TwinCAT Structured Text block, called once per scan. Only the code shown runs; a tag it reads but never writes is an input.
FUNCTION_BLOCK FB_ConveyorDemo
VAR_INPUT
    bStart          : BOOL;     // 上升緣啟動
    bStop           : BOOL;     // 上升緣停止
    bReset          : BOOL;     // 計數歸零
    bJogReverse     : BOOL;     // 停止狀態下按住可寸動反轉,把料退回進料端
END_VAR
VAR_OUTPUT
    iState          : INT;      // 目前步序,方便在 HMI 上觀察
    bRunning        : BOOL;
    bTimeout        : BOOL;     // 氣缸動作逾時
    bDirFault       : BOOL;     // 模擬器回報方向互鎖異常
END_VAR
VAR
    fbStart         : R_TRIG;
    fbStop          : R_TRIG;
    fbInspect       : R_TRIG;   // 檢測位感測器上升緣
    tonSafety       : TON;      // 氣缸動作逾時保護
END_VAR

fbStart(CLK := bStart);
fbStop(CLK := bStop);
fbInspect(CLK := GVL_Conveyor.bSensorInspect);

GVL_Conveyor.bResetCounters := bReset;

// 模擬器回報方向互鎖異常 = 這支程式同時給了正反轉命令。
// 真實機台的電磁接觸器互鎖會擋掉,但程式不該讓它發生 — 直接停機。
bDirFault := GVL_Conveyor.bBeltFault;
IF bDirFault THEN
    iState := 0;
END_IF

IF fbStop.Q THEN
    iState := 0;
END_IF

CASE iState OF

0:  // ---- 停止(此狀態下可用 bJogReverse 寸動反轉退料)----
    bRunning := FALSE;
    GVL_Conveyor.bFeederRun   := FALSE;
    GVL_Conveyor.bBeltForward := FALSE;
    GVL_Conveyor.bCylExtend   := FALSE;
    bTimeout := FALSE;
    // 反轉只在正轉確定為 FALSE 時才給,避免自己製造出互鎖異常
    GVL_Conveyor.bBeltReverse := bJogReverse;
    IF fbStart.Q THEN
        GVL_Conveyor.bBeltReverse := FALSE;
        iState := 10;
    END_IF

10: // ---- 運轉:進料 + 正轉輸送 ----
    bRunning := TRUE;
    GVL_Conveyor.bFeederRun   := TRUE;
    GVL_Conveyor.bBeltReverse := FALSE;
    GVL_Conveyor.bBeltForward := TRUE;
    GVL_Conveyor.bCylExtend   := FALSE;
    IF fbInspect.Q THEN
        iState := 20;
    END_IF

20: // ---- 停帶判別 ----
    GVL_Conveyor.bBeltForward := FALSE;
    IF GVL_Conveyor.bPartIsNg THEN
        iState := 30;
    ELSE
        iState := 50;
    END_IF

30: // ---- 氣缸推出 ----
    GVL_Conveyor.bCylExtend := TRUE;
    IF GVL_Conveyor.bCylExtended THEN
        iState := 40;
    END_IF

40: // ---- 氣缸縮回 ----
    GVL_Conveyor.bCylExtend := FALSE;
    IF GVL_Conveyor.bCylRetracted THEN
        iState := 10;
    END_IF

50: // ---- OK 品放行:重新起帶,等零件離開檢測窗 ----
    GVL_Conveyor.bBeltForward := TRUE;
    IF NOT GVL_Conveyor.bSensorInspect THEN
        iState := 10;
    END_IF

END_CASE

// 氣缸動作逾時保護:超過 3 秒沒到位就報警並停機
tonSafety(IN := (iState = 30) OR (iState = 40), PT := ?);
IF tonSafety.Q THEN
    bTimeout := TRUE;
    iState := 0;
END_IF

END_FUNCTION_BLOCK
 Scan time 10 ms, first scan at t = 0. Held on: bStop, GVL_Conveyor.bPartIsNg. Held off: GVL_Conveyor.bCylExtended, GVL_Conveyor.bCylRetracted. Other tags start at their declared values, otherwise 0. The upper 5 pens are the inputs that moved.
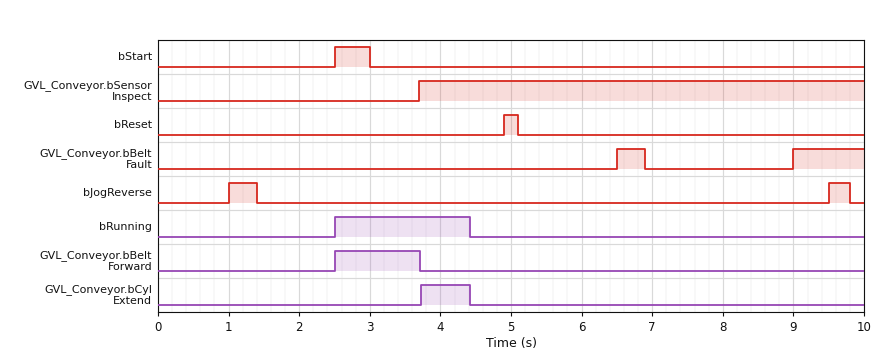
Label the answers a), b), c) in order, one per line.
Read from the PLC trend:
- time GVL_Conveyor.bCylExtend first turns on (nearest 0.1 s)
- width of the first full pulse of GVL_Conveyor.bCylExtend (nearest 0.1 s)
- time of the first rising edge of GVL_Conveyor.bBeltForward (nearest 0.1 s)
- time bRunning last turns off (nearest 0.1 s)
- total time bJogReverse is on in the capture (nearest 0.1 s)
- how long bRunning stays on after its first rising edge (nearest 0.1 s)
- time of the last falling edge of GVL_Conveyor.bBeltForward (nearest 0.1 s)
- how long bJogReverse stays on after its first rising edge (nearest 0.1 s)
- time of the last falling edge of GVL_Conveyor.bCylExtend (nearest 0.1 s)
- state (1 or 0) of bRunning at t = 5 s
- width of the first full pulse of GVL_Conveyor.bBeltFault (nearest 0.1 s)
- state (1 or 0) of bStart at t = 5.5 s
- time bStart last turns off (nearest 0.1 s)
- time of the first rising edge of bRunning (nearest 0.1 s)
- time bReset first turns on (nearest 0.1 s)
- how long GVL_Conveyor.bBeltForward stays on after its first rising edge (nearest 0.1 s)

a) 3.7 s
b) 0.7 s
c) 2.5 s
d) 4.4 s
e) 0.7 s
f) 1.9 s
g) 3.7 s
h) 0.4 s
i) 4.4 s
j) 0
k) 0.4 s
l) 0
m) 3.0 s
n) 2.5 s
o) 4.9 s
p) 1.2 s
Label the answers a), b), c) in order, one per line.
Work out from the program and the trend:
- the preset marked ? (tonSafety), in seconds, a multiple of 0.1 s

a) 0.7 s
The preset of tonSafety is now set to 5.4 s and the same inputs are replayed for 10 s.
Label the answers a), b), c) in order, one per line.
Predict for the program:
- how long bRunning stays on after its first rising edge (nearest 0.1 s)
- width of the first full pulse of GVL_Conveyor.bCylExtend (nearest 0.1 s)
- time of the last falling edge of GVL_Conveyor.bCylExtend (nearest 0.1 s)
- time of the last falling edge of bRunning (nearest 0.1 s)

a) 4.0 s
b) 2.8 s
c) 6.5 s
d) 6.5 s
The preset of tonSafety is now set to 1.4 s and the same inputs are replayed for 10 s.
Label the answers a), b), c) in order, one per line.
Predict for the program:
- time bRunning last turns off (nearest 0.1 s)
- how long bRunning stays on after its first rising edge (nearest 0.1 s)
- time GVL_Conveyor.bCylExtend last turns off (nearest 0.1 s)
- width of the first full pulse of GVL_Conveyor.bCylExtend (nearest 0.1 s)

a) 5.1 s
b) 2.6 s
c) 5.1 s
d) 1.4 s
